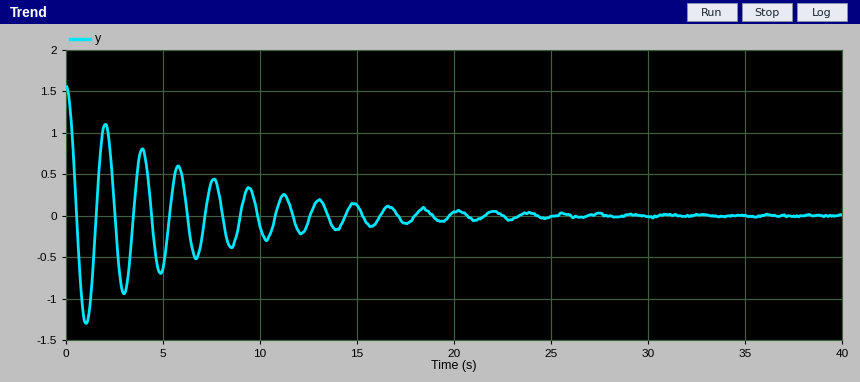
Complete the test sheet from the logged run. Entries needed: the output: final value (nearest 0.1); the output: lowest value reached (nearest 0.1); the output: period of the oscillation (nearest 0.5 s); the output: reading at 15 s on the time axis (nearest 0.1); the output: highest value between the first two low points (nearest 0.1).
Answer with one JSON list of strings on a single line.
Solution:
["0.0", "-1.3", "2.0 s", "0.1", "1.1"]
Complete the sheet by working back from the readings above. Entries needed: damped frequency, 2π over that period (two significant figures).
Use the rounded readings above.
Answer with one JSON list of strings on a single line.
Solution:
["3.1 rad/s"]
